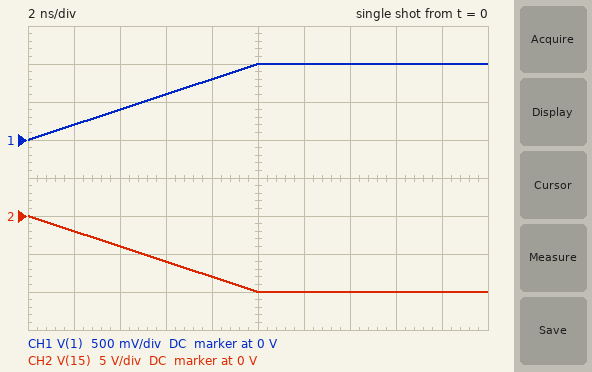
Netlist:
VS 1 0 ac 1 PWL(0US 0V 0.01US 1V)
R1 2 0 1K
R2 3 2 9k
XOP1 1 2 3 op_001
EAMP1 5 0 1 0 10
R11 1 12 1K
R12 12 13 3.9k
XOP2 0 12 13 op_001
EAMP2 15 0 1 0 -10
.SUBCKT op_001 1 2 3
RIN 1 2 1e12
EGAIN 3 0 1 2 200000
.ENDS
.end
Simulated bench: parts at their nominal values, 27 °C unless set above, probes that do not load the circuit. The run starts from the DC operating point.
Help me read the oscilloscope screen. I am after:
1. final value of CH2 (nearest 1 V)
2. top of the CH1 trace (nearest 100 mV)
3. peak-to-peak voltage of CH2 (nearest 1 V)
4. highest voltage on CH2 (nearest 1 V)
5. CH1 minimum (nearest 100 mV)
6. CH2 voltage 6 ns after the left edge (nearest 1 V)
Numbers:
-10 V
1.0 V
10 V
0 V
0 V
-6 V
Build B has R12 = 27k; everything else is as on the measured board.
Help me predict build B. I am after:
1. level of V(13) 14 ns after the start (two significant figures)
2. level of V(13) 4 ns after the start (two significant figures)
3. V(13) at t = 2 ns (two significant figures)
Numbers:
-27 V
-11 V
-5.4 V
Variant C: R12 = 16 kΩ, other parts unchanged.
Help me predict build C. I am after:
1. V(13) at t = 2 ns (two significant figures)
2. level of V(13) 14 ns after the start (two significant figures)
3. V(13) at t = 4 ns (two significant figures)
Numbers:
-3.2 V
-16 V
-6.4 V
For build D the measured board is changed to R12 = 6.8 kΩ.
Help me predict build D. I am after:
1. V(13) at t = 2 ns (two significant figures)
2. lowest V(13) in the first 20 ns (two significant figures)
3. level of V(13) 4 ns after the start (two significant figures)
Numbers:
-1.4 V
-6.8 V
-2.7 V
